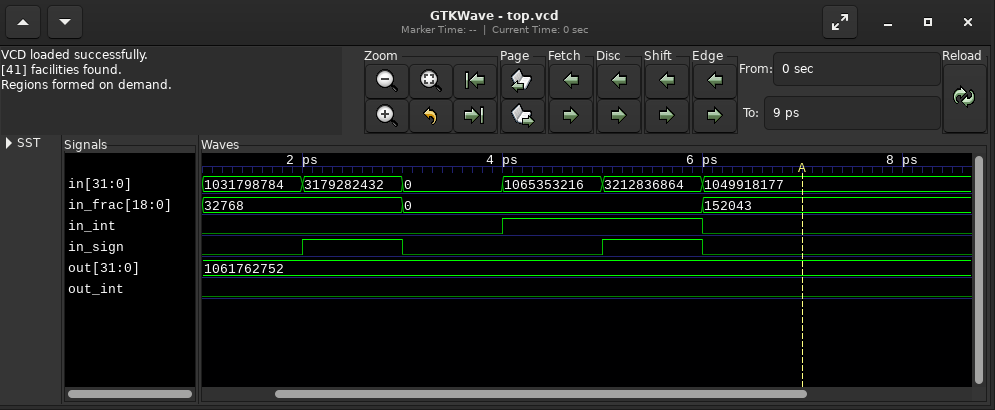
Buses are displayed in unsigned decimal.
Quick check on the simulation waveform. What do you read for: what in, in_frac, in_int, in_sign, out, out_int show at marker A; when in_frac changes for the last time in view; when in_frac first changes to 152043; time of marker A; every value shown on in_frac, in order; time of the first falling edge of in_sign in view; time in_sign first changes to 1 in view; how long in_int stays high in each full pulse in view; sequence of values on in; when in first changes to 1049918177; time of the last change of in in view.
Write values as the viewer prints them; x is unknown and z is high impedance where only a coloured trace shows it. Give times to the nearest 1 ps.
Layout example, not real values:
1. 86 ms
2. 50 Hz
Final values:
1. in=1049918177, in_frac=152043, in_int=0, in_sign=0, out=1061762752, out_int=0
2. 6 ps
3. 6 ps
4. 7 ps
5. 32768, 0, 152043
6. 3 ps
7. 2 ps
8. 2 ps
9. 1031798784, 3179282432, 0, 1065353216, 3212836864, 1049918177
10. 6 ps
11. 6 ps
